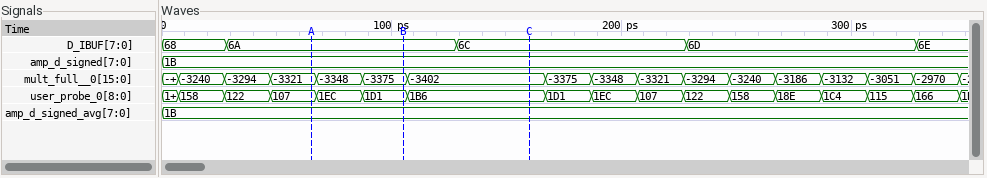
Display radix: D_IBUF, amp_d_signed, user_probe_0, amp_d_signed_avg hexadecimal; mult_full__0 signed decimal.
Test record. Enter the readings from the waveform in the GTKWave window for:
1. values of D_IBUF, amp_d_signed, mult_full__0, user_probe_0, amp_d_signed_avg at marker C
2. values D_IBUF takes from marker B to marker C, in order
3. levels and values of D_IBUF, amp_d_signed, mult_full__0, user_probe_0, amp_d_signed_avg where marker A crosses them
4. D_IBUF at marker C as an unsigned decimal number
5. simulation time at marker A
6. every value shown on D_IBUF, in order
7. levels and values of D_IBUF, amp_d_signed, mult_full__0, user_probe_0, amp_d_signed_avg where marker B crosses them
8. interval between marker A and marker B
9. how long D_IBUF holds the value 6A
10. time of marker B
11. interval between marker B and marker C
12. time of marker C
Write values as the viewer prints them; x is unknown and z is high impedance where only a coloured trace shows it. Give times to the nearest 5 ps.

D_IBUF=6C, amp_d_signed=1B, mult_full__0=-3402, user_probe_0=1B6, amp_d_signed_avg=1B
6A, 6C
D_IBUF=6A, amp_d_signed=1B, mult_full__0=-3321, user_probe_0=107, amp_d_signed_avg=1B
108
65 ps
68, 6A, 6C, 6D, 6E
D_IBUF=6A, amp_d_signed=1B, mult_full__0=-3375, user_probe_0=1D1, amp_d_signed_avg=1B
40 ps
100 ps
105 ps
55 ps
160 ps
